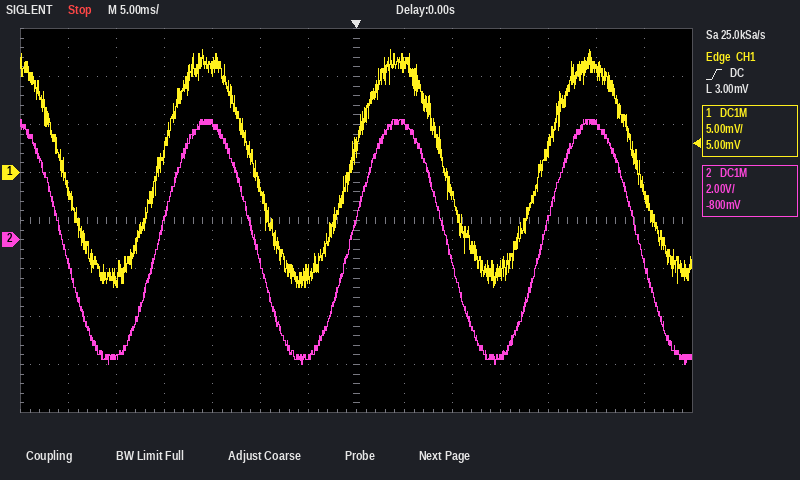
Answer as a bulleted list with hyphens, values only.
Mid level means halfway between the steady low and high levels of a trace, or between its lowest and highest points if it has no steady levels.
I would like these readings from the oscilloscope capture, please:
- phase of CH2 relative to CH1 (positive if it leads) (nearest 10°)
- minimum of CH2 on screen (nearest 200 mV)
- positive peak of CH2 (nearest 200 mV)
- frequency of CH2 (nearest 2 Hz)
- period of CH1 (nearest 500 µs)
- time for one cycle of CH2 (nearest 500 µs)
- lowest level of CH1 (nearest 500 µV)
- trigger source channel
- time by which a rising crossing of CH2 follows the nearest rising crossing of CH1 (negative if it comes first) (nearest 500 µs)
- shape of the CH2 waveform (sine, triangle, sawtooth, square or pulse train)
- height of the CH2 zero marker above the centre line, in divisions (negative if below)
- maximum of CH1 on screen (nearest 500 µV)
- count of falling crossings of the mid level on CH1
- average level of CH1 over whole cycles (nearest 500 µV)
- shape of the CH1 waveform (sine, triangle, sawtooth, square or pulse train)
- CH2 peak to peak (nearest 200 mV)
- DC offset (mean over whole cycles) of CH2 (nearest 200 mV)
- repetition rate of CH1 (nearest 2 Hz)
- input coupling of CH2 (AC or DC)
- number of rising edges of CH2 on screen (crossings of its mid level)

- 0°
- -5.2 V
- 5.0 V
- 50 Hz
- 20.0 ms
- 20.0 ms
- -12.0 mV
- CH1
- 0.0 ms
- sine
- -0.4 div
- 13.0 mV
- 4
- 500 µV
- sine
- 10.2 V
- 0.0 V
- 50 Hz
- DC
- 3
